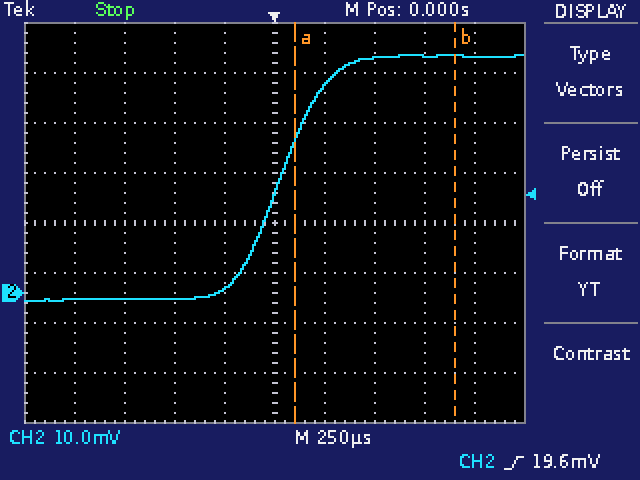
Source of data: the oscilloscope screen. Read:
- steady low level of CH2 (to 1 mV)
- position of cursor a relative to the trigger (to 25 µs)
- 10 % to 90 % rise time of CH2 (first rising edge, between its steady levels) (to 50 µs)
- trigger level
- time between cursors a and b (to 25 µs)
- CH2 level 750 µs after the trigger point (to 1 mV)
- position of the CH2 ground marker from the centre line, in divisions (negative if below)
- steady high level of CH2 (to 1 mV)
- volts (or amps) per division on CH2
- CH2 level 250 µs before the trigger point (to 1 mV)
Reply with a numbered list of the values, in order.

1. -1 mV
2. +100 µs
3. 450 µs
4. 19.6 mV
5. 800 µs
6. 47 mV
7. -1.4 div
8. 47 mV
9. 10 mV
10. 1 mV
